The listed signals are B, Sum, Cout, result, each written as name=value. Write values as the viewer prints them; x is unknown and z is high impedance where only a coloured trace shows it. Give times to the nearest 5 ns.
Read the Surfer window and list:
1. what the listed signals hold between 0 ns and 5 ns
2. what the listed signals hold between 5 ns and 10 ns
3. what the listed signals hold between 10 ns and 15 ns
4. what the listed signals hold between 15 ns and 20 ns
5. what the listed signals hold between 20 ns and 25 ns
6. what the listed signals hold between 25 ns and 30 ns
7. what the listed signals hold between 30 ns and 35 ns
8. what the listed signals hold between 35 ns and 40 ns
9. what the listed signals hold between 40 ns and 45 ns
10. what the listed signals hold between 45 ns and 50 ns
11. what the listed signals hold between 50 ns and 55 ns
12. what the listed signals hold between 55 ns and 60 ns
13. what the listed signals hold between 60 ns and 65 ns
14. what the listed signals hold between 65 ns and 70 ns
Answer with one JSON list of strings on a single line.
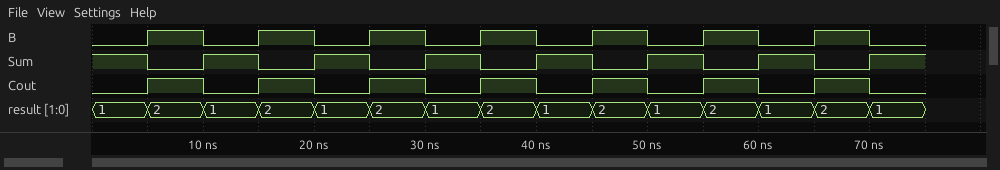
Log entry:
["B=0, Sum=1, Cout=0, result=1", "B=1, Sum=0, Cout=1, result=2", "B=0, Sum=1, Cout=0, result=1", "B=1, Sum=0, Cout=1, result=2", "B=0, Sum=1, Cout=0, result=1", "B=1, Sum=0, Cout=1, result=2", "B=0, Sum=1, Cout=0, result=1", "B=1, Sum=0, Cout=1, result=2", "B=0, Sum=1, Cout=0, result=1", "B=1, Sum=0, Cout=1, result=2", "B=0, Sum=1, Cout=0, result=1", "B=1, Sum=0, Cout=1, result=2", "B=0, Sum=1, Cout=0, result=1", "B=1, Sum=0, Cout=1, result=2"]
